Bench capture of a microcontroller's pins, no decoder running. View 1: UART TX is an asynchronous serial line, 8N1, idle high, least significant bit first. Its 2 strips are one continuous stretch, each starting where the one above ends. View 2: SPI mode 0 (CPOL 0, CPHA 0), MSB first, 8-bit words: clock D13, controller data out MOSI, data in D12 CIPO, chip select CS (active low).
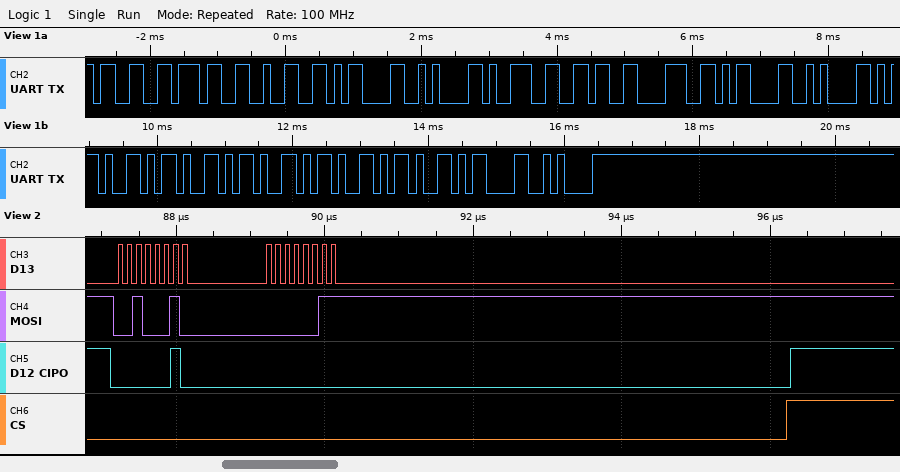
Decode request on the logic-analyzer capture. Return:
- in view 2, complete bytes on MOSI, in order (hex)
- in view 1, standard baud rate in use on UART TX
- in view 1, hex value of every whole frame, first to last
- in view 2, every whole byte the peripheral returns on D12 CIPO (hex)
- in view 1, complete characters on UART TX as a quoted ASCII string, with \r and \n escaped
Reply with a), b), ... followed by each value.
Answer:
a) 22 03
b) 9600 baud
c) 0x33 0x37 0x32 0x0D 0x0A 0x39 0x36 0x38 0x0D 0x0A 0x2D 0x2D 0x2D 0x2D 0x2D 0x0D 0x0A
d) 02 00
e) "372\r\n968\r\n-----\r\n"
